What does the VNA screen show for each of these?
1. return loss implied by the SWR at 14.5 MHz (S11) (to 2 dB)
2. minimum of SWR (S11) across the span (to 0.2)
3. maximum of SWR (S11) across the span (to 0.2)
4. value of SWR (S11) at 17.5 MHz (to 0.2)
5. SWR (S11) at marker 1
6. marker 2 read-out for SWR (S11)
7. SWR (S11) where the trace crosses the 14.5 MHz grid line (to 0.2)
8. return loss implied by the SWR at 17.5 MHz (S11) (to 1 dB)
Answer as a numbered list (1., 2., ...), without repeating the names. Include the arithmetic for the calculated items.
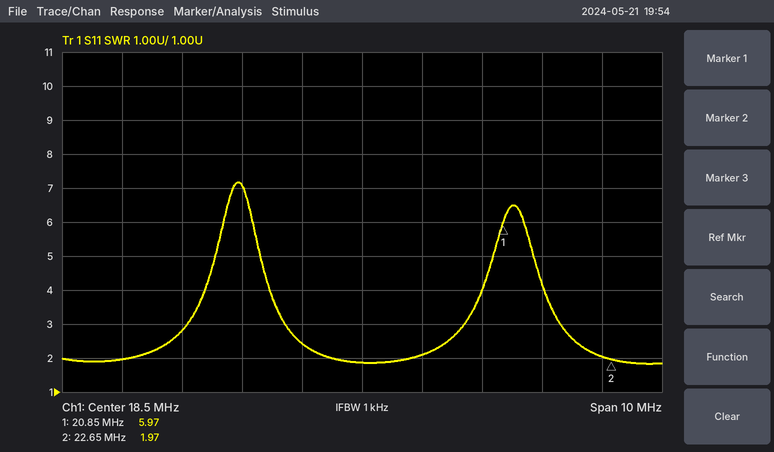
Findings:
1. −20 log10((2 − 1)/(2 + 1)) ≈ 10 dB
2. 1.8
3. 7.2
4. 2.4
5. 5.97
6. 1.97
7. 2.0
8. −20 log10((2.4 − 1)/(2.4 + 1)) ≈ 8 dB
